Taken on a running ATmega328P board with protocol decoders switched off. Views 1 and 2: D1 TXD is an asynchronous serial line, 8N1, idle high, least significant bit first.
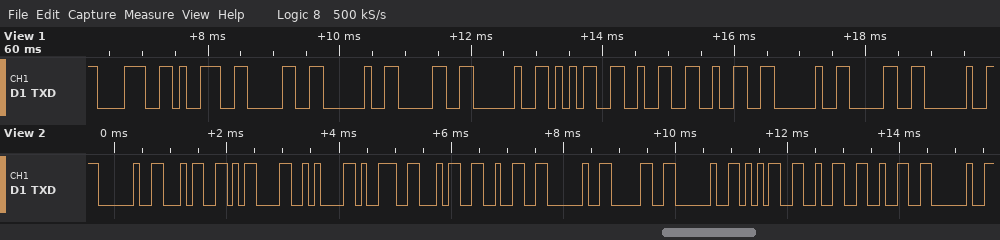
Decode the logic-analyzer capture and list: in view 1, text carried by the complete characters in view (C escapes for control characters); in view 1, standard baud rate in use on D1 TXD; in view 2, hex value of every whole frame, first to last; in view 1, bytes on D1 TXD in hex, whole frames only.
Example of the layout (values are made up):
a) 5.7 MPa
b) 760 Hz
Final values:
a) "890 0 522 0 "
b) 9600 baud
c) 0x20 0x34 0x0D 0x0A 0x39 0x34 0x32 0x20 0x30 0x20 0x35 0x32 0x32 0x20
d) 38 39 30 20 30 20 35 32 32 20 30 20
